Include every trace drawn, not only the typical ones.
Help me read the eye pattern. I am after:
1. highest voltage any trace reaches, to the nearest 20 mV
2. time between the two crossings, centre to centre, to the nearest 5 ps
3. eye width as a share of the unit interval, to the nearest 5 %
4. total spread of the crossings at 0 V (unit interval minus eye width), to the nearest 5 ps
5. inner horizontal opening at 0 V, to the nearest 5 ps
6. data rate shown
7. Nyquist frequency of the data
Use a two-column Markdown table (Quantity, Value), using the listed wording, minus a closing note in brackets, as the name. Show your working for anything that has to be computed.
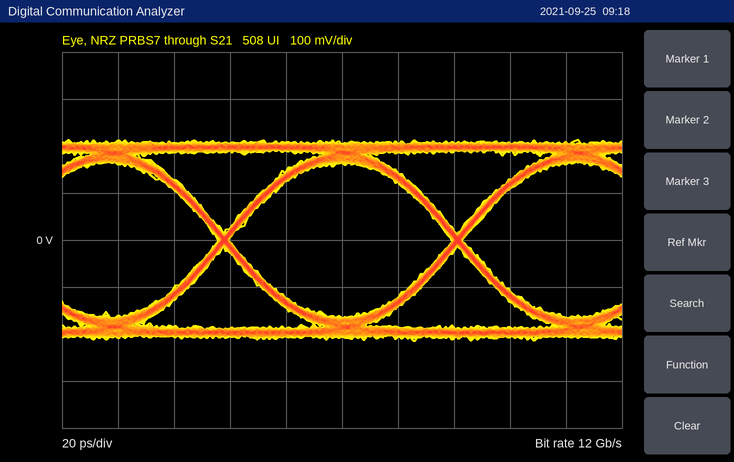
| Quantity | Value |
|---|---|
| highest voltage any trace reaches, to the nearest 20 mV | 220 mV |
| time between the two crossings, centre to centre, to the nearest 5 ps | 85 ps |
| eye width as a share of the unit interval, to the nearest 5 % | 80 ps / 85 ps ≈ 94.1 %, so 95 % to the nearest 5 % |
| total spread of the crossings at 0 V (unit interval minus eye width), to the nearest 5 ps | 5 ps |
| inner horizontal opening at 0 V, to the nearest 5 ps | 80 ps |
| data rate shown | 12 Gb/s |
| Nyquist frequency of the data | 6 GHz |
